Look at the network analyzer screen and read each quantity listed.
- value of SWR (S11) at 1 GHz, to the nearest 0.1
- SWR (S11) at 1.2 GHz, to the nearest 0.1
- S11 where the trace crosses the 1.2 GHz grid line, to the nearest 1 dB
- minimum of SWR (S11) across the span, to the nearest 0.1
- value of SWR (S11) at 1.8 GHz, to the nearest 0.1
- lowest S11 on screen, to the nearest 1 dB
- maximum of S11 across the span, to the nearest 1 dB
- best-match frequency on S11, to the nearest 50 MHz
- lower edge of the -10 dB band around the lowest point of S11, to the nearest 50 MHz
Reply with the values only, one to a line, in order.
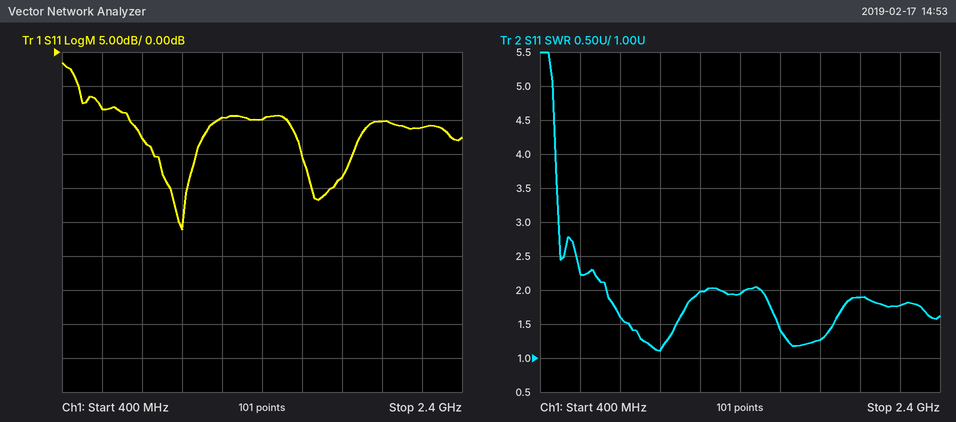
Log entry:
1.1
2.0
-10 dB
1.1
1.3
-26 dB
-2 dB
1.00 GHz
750 MHz
